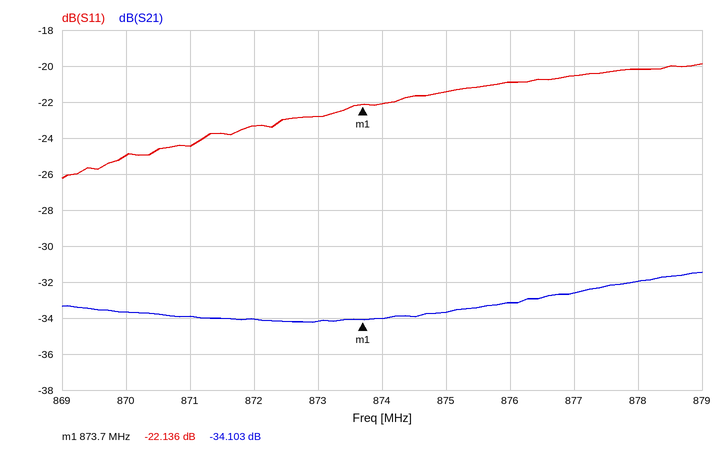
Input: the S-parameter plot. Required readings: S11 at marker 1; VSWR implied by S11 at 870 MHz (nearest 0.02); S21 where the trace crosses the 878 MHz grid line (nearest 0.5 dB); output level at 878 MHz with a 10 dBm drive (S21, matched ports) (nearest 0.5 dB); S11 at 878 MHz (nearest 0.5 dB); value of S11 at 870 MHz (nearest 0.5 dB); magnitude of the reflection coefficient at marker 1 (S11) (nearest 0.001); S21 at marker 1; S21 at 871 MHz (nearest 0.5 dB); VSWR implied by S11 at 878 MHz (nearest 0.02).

-22.136 dB
1.12
-32.0 dB
-22.0 dBm
-20.0 dB
-25.0 dB
0.078
-34.103 dB
-34.0 dB
1.22
